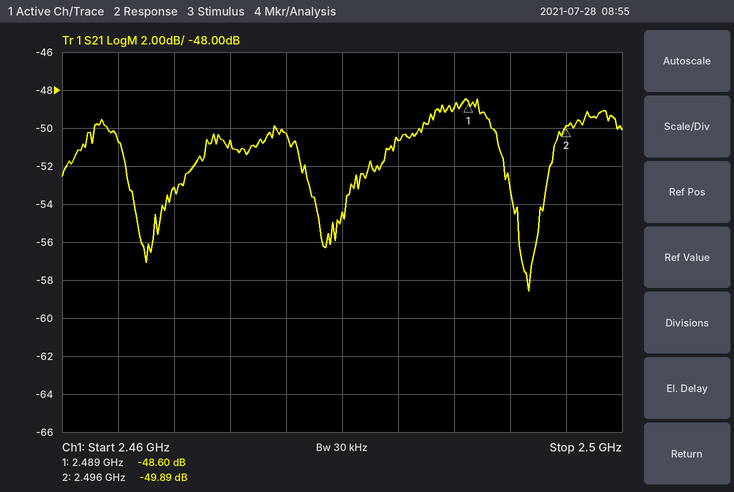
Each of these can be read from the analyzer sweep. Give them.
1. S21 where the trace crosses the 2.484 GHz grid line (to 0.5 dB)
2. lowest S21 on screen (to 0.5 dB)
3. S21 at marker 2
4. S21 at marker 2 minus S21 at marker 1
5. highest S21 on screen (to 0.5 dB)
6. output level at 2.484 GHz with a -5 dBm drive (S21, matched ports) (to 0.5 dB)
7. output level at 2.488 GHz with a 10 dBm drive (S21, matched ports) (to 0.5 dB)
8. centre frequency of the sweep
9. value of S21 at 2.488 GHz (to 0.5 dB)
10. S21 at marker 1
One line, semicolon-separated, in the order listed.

-50.5 dB; -58.5 dB; -49.89 dB; -1.29 dB; -48.5 dB; -55.5 dBm; -39.0 dBm; 2.48 GHz; -49.0 dB; -48.60 dB
